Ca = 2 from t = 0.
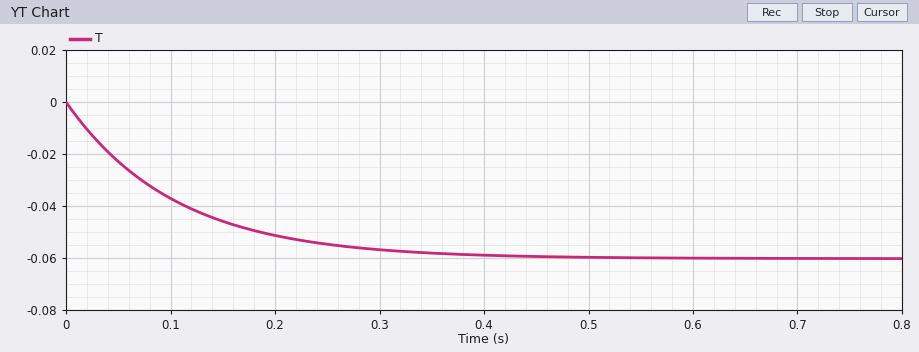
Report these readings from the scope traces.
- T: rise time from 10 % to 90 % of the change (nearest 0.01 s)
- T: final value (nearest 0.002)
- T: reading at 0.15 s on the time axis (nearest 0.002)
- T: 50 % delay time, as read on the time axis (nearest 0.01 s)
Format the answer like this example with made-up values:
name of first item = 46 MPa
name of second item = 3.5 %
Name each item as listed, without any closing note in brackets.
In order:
T: rise time from 10 % to 90 % of the change = 0.23 s
T: final value = -0.060
T: reading at 0.15 s on the time axis = -0.046
T: 50 % delay time, as read on the time axis = 0.07 s
